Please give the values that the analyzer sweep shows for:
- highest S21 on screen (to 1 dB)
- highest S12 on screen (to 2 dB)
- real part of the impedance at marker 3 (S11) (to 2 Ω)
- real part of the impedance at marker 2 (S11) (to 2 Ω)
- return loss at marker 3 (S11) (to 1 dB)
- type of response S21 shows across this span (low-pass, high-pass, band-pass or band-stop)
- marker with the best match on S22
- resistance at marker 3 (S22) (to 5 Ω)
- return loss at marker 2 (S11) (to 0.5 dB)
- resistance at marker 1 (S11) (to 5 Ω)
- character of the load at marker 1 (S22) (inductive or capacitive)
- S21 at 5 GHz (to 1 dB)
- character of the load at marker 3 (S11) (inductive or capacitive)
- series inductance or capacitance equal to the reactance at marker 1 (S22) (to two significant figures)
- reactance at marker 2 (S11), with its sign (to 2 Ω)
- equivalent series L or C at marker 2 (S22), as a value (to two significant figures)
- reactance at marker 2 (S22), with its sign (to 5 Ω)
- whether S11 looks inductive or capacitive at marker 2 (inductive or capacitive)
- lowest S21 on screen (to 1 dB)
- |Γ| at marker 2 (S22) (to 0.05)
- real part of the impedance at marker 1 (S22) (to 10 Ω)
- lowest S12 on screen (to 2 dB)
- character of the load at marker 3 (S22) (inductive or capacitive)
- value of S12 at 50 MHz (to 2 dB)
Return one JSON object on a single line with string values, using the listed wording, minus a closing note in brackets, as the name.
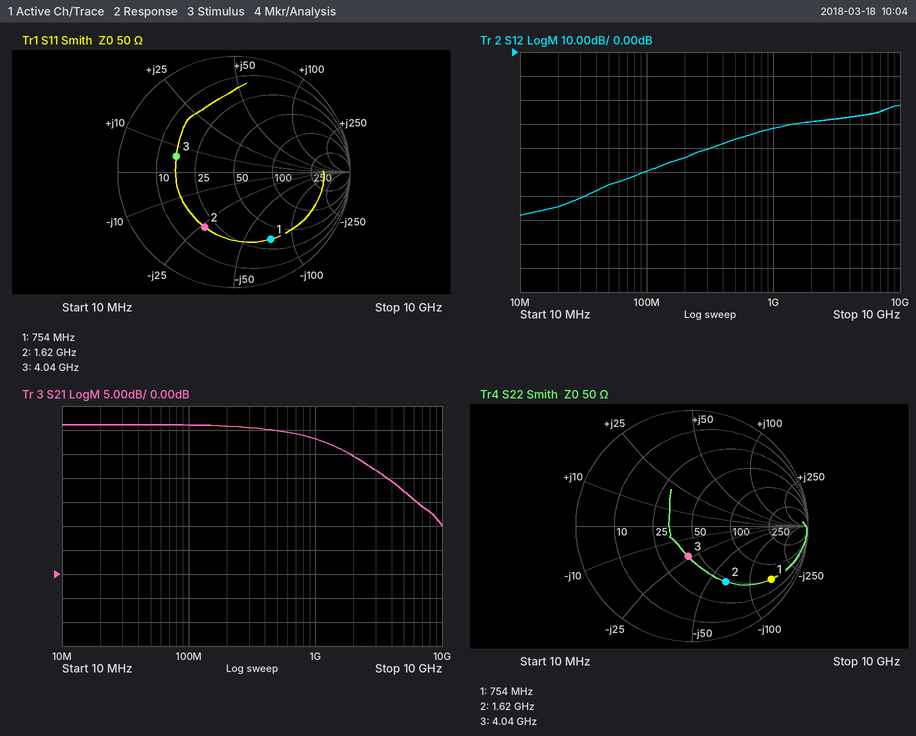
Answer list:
{"highest S21 on screen": "31 dB", "highest S12 on screen": "-22 dB", "real part of the impedance at marker 3 (S11)": "16 Ω", "real part of the impedance at marker 2 (S11)": "20 Ω", "return loss at marker 3 (S11)": "6 dB", "type of response S21 shows across this span": "low-pass", "marker with the best match on S22": "marker 3", "resistance at marker 3 (S22)": "40 Ω", "return loss at marker 2 (S11)": "5.5 dB", "resistance at marker 1 (S11)": "35 Ω", "character of the load at marker 1 (S22)": "capacitive", "S21 at 5 GHz": "17 dB", "character of the load at marker 3 (S11)": "inductive", "series inductance or capacitance equal to the reactance at marker 1 (S22)": "1.4 pF", "reactance at marker 2 (S11), with its sign": "-26 Ω", "equivalent series L or C at marker 2 (S22), as a value": "1.5 pF", "reactance at marker 2 (S22), with its sign": "-65 Ω", "whether S11 looks inductive or capacitive at marker 2": "capacitive", "lowest S21 on screen": "10 dB", "|Γ| at marker 2 (S22)": "0.55", "real part of the impedance at marker 1 (S22)": "50 Ω", "lowest S12 on screen": "-68 dB", "character of the load at marker 3 (S22)": "capacitive", "value of S12 at 50 MHz": "-56 dB"}
